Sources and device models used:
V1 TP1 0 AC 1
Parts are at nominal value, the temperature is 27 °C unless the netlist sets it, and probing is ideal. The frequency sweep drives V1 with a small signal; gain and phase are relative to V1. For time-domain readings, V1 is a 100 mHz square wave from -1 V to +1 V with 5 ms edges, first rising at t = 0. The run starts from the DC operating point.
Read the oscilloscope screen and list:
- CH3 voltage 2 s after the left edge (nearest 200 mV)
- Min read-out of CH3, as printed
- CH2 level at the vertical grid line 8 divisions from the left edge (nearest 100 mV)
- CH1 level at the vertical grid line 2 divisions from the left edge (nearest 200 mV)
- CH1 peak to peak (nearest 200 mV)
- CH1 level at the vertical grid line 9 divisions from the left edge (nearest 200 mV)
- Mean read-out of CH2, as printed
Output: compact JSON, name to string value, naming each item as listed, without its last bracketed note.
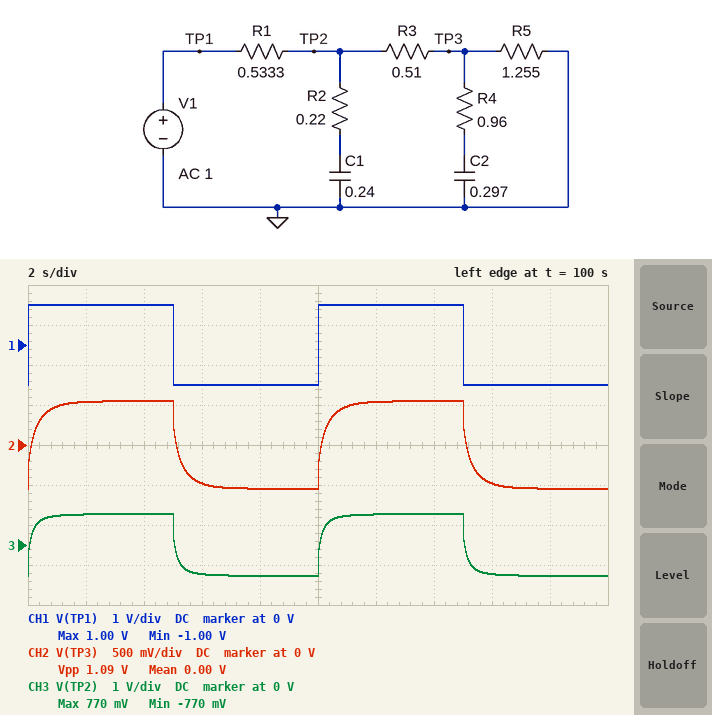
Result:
{"CH3 voltage 2 s after the left edge": "800 mV", "Min read-out of CH3, as printed": "-770 mV", "CH2 level at the vertical grid line 8 divisions from the left edge": "-500 mV", "CH1 level at the vertical grid line 2 divisions from the left edge": "1.0 V", "CH1 peak to peak": "2.0 V", "CH1 level at the vertical grid line 9 divisions from the left edge": "-1.0 V", "Mean read-out of CH2, as printed": "0.00 V"}
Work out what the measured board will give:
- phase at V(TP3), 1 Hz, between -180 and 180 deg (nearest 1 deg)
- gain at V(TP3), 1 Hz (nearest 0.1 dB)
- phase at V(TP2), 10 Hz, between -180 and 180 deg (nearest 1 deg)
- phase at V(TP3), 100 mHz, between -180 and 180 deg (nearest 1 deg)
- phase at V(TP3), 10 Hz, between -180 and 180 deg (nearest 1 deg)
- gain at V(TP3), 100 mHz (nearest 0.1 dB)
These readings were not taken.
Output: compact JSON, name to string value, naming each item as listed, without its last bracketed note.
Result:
{"phase at V(TP3), 1 Hz, between -180 and 180 deg": "-32 deg", "gain at V(TP3), 1 Hz": "-10.8 dB", "phase at V(TP2), 10 Hz, between -180 and 180 deg": "-10 deg", "phase at V(TP3), 100 mHz, between -180 and 180 deg": "-9 deg", "phase at V(TP3), 10 Hz, between -180 and 180 deg": "-11 deg", "gain at V(TP3), 100 mHz": "-5.5 dB"}
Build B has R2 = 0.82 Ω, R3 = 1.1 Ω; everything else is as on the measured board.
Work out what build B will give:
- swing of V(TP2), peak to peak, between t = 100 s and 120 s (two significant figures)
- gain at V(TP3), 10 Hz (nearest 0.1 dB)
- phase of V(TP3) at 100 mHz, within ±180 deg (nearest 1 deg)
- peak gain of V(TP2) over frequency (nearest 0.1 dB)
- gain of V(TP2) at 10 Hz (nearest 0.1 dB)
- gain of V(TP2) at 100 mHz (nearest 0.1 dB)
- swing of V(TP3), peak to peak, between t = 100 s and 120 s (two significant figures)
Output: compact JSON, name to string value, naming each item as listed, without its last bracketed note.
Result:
{"swing of V(TP2), peak to peak, between t = 100 s and 120 s": "1.6 V", "gain at V(TP3), 10 Hz": "-15.5 dB", "phase of V(TP3) at 100 mHz, within ±180 deg": "-11 deg", "peak gain of V(TP2) over frequency": "-1.8 dB", "gain of V(TP2) at 10 Hz": "-5.9 dB", "gain of V(TP2) at 100 mHz": "-1.9 dB", "swing of V(TP3), peak to peak, between t = 100 s and 120 s": "870 mV"}
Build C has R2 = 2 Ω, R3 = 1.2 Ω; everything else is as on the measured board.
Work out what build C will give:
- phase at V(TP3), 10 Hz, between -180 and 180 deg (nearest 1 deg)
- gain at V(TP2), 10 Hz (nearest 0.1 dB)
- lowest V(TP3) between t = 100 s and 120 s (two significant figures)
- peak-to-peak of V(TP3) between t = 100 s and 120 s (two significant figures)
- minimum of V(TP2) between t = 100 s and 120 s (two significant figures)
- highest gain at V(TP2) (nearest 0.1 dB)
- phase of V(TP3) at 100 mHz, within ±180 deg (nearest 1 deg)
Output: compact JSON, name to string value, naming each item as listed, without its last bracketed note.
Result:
{"phase at V(TP3), 10 Hz, between -180 and 180 deg": "-2 deg", "gain at V(TP2), 10 Hz": "-3.9 dB", "lowest V(TP3) between t = 100 s and 120 s": "-420 mV", "peak-to-peak of V(TP3) between t = 100 s and 120 s": "840 mV", "minimum of V(TP2) between t = 100 s and 120 s": "-820 mV", "highest gain at V(TP2)": "-1.7 dB", "phase of V(TP3) at 100 mHz, within ±180 deg": "-11 deg"}
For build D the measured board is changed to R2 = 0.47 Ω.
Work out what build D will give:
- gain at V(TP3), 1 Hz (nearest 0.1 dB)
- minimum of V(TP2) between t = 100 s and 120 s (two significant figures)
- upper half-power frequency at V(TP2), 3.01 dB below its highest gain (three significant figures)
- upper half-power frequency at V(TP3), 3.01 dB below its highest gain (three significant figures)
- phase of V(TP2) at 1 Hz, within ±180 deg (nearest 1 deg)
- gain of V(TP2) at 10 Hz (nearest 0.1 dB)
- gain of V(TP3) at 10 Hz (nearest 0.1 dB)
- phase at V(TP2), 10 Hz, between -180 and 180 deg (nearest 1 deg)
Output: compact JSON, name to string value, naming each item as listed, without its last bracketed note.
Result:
{"gain at V(TP3), 1 Hz": "-11.0 dB", "minimum of V(TP2) between t = 100 s and 120 s": "-770 mV", "upper half-power frequency at V(TP2), 3.01 dB below its highest gain": "816 mHz", "upper half-power frequency at V(TP3), 3.01 dB below its highest gain": "453 mHz", "phase of V(TP2) at 1 Hz, within ±180 deg": "-18 deg", "gain of V(TP2) at 10 Hz": "-8.4 dB", "gain of V(TP3) at 10 Hz": "-14.1 dB", "phase at V(TP2), 10 Hz, between -180 and 180 deg": "-4 deg"}
